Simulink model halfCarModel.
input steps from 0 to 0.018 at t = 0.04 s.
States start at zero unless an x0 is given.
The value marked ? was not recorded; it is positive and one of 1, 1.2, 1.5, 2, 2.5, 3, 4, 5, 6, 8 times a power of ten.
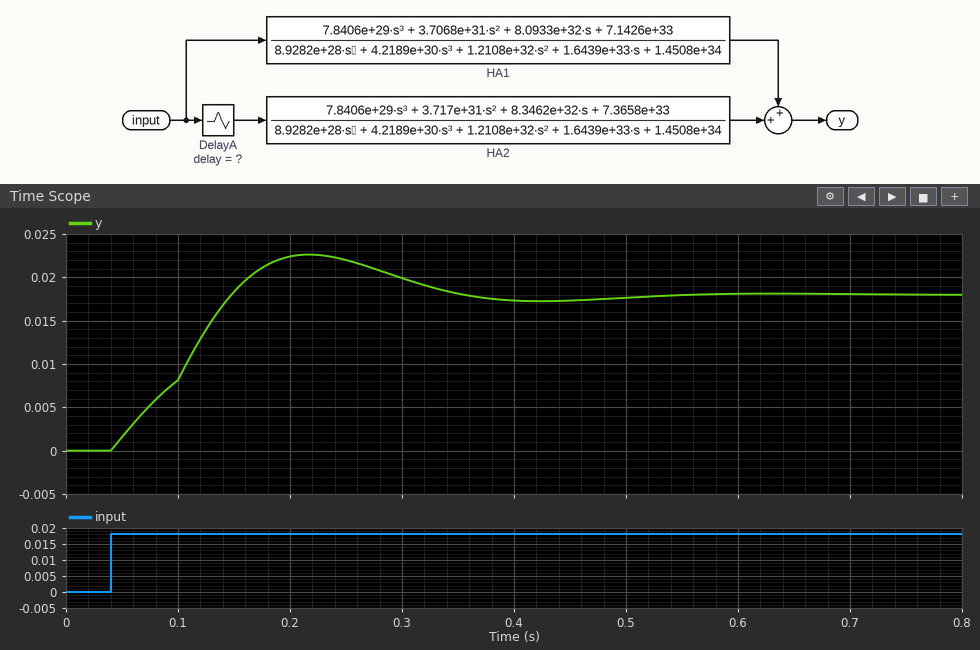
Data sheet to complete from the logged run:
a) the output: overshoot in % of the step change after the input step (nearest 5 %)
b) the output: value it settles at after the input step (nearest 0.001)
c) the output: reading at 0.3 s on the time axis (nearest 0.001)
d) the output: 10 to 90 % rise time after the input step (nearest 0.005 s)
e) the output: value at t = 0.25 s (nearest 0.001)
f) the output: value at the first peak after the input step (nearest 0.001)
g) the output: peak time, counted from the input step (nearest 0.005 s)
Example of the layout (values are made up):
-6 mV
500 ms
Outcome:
25 %
0.018
0.020
0.085 s
0.022
0.023
0.175 s
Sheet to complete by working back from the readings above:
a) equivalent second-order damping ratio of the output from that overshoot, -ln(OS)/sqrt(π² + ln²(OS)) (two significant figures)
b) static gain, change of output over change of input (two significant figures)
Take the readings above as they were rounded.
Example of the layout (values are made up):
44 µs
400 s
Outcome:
0.40
1.0
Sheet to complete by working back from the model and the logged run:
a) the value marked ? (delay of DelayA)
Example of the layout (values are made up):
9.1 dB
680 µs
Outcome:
0.06
